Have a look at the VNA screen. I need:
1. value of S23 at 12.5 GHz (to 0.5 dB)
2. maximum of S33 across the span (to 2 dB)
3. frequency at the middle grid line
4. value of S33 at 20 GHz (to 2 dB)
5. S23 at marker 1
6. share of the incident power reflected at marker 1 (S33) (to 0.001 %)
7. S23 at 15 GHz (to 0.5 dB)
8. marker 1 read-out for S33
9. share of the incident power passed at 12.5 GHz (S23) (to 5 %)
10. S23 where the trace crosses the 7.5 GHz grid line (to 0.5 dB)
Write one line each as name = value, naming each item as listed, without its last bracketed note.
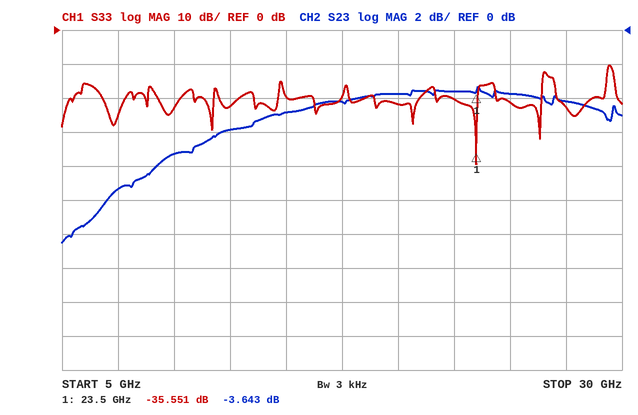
value of S23 at 12.5 GHz = -6.0 dB
maximum of S33 across the span = -10 dB
frequency at the middle grid line = 17.5 GHz
value of S33 at 20 GHz = -22 dB
S23 at marker 1 = -3.643 dB
share of the incident power reflected at marker 1 (S33) = 0.028 %
S23 at 15 GHz = -5.0 dB
marker 1 read-out for S33 = -35.551 dB
share of the incident power passed at 12.5 GHz (S23) = 25 %
S23 where the trace crosses the 7.5 GHz grid line = -9.5 dB
